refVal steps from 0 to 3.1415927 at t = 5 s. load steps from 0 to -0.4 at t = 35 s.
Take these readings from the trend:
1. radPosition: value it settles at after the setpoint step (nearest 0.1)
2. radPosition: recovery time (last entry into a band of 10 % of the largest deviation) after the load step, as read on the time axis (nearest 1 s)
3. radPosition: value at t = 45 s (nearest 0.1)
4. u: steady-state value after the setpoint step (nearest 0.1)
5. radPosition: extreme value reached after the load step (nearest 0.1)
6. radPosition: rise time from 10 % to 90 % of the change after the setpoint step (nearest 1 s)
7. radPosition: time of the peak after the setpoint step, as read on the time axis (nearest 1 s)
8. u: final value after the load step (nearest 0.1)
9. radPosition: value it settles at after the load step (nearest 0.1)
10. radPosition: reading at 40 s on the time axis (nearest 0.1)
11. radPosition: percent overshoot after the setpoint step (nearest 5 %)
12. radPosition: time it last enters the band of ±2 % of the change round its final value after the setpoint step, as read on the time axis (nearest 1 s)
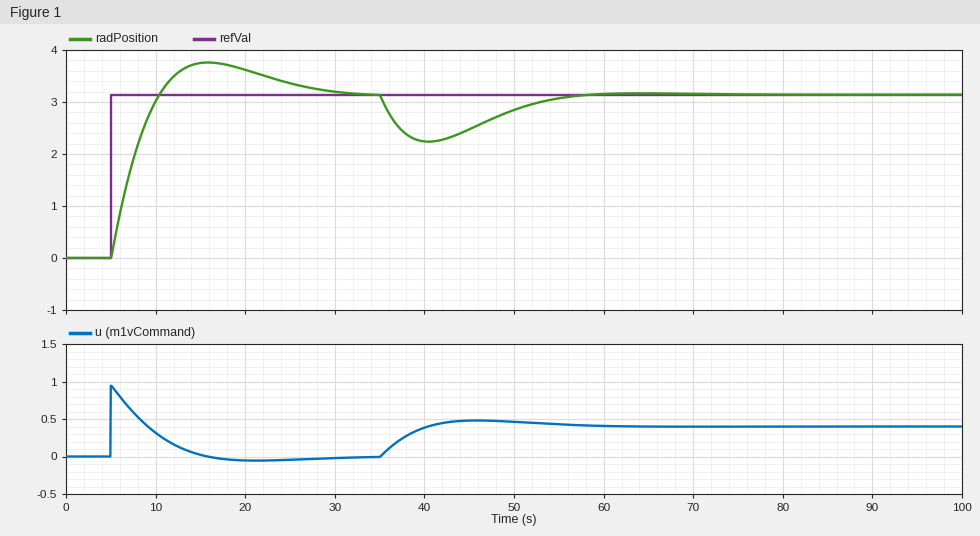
3.1
54 s
2.5
0.0
2.2
4 s
16 s
0.4
3.1
2.2
20 %
30 s
